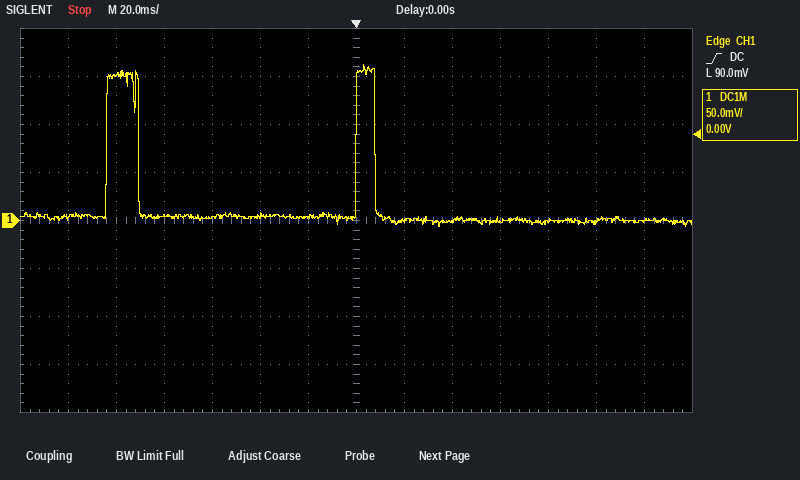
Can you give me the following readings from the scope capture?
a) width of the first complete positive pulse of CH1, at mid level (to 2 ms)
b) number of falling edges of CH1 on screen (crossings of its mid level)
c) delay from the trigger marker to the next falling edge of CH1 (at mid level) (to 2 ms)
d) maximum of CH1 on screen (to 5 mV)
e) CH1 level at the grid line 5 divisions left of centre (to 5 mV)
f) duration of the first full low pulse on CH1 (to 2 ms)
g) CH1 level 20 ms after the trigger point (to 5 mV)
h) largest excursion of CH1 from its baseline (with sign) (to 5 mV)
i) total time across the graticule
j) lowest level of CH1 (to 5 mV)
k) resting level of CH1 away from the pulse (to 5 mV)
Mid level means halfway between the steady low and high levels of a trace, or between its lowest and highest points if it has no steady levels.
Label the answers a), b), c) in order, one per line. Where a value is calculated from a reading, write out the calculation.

a) 14 ms
b) 2
c) 8 ms
d) 160 mV
e) 150 mV
f) 90 ms
g) 0 mV
h) 160 mV − (0 mV) = +160 mV
i) 280 ms
j) -5 mV
k) 0 mV
